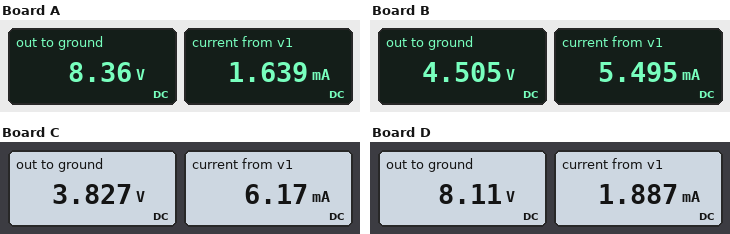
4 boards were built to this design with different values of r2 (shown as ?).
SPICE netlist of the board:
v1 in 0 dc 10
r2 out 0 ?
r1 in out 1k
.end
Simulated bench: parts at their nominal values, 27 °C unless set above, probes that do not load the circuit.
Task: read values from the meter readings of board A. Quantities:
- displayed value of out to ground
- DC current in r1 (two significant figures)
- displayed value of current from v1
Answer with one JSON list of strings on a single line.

["8.36 V", "1.6 mA", "1.639 mA"]
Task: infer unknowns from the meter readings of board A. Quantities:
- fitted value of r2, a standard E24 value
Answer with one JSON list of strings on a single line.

["5.1 kΩ"]
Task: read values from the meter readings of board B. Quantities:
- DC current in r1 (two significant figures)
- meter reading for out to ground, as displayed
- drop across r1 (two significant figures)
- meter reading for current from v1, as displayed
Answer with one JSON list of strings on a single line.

["5.5 mA", "4.505 V", "5.5 V", "5.495 mA"]
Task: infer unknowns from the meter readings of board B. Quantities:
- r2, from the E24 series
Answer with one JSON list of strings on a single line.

["820 Ω"]
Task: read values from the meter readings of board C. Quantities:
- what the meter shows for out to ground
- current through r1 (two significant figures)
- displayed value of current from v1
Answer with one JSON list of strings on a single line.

["3.827 V", "6.2 mA", "6.17 mA"]
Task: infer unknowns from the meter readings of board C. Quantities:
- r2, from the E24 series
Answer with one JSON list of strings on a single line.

["620 Ω"]
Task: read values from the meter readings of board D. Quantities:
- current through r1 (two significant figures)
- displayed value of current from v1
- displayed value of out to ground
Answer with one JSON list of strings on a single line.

["1.9 mA", "1.887 mA", "8.11 V"]
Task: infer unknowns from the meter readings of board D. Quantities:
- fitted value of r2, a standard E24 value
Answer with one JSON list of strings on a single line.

["4.3 kΩ"]
